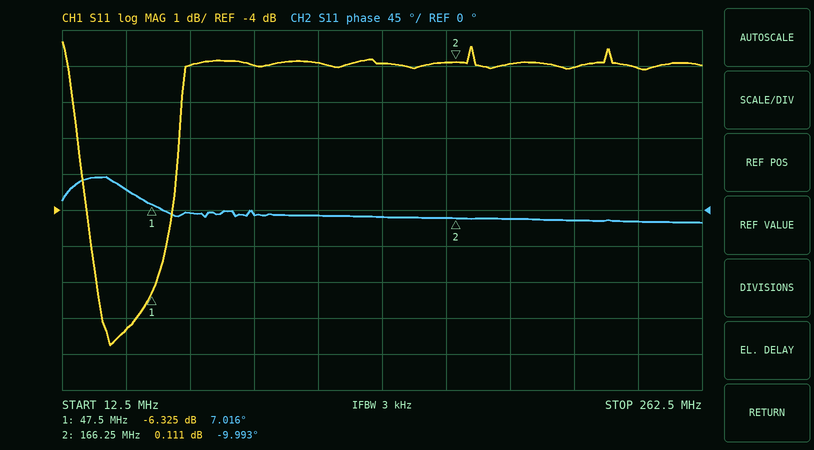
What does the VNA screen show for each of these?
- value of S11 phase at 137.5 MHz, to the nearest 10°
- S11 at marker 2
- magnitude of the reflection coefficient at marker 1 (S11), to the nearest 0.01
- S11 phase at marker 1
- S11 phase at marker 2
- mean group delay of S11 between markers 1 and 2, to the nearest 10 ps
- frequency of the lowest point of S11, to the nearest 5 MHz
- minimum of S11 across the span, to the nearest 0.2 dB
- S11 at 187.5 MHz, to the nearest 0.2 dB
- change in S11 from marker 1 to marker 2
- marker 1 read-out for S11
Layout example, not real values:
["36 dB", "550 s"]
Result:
["-10°", "0.111 dB", "0.48", "7.016°", "-9.993°", "400 ps", "30 MHz", "-7.8 dB", "0.0 dB", "6.436 dB", "-6.325 dB"]
